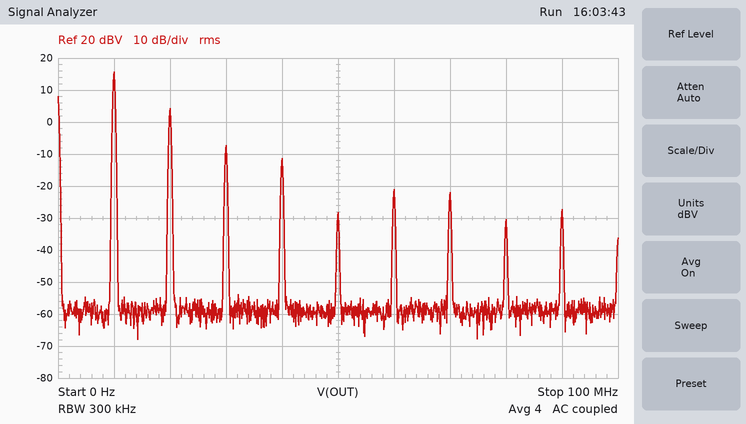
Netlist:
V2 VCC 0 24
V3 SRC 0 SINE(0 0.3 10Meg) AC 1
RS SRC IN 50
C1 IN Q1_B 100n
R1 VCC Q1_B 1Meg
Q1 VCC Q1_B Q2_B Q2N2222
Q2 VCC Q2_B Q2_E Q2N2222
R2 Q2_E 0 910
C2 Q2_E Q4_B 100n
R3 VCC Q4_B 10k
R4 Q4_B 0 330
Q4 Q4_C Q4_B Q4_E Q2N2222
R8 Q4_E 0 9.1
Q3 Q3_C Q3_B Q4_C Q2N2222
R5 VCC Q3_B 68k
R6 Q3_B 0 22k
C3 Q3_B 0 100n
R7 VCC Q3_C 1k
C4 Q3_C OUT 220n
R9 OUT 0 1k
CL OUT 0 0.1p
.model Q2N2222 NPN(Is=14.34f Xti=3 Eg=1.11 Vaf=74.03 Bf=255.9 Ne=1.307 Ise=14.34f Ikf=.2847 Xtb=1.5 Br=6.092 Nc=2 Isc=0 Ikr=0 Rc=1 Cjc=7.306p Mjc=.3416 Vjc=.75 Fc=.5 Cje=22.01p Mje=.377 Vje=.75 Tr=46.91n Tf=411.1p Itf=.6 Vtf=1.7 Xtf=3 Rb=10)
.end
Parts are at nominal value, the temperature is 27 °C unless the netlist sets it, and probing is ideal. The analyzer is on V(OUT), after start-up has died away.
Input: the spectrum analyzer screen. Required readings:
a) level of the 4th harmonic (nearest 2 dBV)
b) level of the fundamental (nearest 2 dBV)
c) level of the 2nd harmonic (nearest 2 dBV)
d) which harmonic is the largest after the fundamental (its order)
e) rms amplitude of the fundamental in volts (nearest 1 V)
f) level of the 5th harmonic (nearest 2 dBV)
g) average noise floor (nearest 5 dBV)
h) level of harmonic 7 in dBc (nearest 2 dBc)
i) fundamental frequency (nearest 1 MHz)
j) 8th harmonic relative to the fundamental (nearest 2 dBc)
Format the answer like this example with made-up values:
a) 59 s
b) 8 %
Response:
a) -12 dBV
b) 16 dBV
c) 4 dBV
d) 2
e) 6 V
f) -28 dBV
g) -60 dBV
h) -38 dBc
i) 10 MHz
j) -46 dBc
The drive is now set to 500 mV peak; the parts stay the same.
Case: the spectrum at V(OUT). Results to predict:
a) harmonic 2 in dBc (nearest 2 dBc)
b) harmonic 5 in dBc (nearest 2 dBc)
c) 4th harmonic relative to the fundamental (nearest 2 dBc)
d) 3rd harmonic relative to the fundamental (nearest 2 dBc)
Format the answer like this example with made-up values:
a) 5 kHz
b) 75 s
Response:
a) -16 dBc
b) -22 dBc
c) -18 dBc
d) -12 dBc
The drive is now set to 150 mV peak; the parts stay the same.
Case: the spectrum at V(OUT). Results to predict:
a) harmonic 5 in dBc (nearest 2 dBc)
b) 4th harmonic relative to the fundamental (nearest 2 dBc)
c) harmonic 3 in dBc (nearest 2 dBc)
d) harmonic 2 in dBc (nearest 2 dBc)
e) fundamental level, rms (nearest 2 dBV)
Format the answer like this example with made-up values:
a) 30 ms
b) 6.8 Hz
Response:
a) -52 dBc
b) -48 dBc
c) -28 dBc
d) -16 dBc
e) 10 dBV
